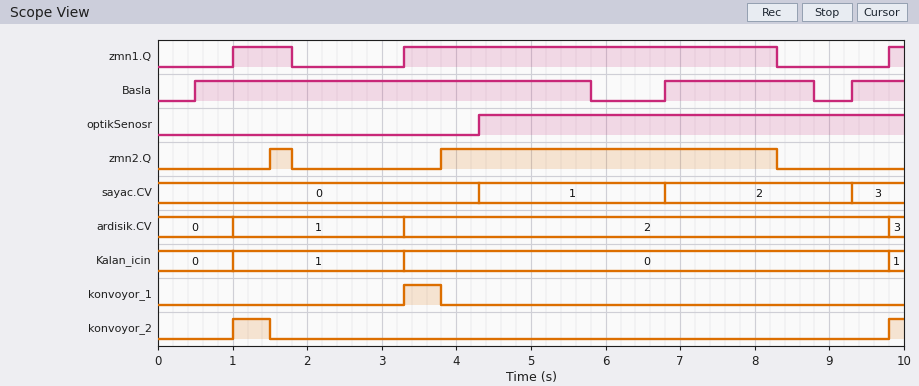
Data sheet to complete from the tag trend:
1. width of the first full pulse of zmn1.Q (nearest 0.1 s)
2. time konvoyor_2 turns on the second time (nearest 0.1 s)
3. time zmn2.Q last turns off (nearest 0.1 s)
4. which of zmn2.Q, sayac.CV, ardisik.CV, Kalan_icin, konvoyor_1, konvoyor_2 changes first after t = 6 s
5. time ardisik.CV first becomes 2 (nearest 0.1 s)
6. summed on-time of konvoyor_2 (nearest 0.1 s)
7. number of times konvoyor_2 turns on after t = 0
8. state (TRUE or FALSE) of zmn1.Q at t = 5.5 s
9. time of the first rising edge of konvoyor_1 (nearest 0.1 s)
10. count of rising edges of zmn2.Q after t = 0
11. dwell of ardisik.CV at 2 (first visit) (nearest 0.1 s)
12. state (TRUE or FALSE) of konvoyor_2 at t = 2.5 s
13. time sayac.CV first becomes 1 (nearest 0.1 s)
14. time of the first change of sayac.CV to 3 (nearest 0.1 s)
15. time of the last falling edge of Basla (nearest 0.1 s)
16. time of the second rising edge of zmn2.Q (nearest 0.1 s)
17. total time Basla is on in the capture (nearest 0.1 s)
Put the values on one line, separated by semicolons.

0.8 s; 9.8 s; 8.3 s; sayac.CV; 3.3 s; 0.7 s; 2; TRUE; 3.3 s; 2; 6.5 s; FALSE; 4.3 s; 9.3 s; 8.8 s; 3.8 s; 8.0 s
